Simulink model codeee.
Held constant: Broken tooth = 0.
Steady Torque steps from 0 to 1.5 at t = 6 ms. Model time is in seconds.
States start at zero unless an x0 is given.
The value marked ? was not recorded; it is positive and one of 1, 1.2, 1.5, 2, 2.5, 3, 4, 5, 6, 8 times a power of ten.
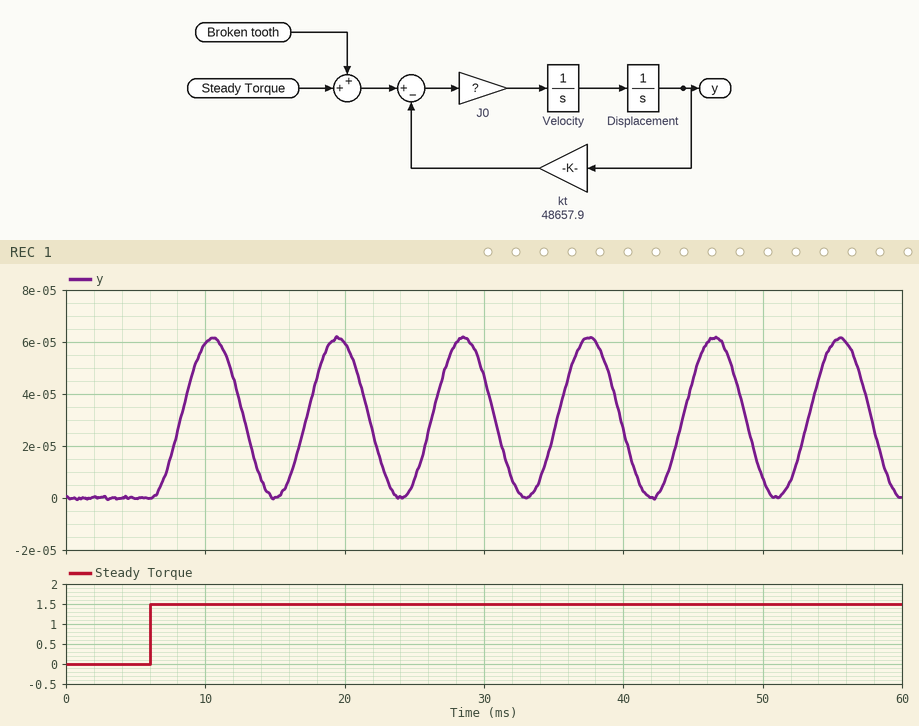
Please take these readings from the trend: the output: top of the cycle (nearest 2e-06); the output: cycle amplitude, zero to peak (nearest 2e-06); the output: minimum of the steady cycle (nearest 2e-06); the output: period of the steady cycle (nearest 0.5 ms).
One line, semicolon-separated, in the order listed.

0.000062; 0.000030; 0.000000; 9.0 ms
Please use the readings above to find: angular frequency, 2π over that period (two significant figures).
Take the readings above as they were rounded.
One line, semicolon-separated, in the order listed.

0.70 rad/ms
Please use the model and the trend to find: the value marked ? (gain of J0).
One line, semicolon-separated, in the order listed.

10
